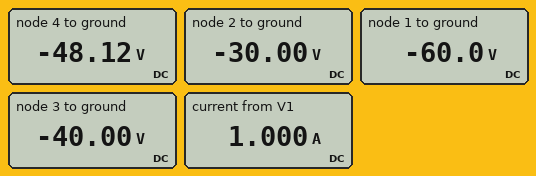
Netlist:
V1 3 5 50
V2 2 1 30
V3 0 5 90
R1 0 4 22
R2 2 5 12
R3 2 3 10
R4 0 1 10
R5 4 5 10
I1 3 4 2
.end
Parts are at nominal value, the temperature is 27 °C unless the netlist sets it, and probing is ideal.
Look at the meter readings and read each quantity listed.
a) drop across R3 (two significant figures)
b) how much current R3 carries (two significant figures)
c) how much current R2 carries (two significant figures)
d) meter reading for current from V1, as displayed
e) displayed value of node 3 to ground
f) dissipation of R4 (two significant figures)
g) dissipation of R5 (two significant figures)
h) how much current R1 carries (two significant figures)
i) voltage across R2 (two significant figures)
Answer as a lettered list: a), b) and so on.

a) 10 V
b) 1.0 A
c) 5.0 A
d) 1.000 A
e) -40.00 V
f) 360 W
g) 180 W
h) 2.2 A
i) 60 V
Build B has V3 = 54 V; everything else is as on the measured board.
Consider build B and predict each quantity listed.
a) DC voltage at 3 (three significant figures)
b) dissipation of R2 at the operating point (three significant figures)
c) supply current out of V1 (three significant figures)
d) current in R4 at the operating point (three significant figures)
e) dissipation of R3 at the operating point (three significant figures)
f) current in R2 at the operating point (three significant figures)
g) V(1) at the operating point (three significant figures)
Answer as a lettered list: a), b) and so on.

a) -4.00 V
b) 186 W
c) 2.27 A
d) 3.67 A
e) 732 mW
f) 3.94 A
g) -36.7 V
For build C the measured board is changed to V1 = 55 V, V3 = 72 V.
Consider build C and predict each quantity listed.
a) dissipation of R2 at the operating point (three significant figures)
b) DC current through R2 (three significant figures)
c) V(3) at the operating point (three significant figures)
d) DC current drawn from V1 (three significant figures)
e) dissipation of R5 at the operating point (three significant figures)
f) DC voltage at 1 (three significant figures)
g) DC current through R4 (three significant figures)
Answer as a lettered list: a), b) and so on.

a) 256 W
b) 4.62 A
c) -17.0 V
d) 1.96 A
e) 131 W
f) -46.6 V
g) 4.66 A
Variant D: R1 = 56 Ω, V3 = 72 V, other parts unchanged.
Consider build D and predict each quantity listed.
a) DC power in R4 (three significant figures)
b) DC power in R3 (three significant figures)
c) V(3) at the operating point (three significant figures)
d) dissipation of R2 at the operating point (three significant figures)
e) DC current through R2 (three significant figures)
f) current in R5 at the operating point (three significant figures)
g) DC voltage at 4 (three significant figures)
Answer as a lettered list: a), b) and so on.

a) 234 W
b) 1.33 W
c) -22.0 V
d) 240 W
e) 4.47 A
f) 2.79 A
g) -44.1 V
